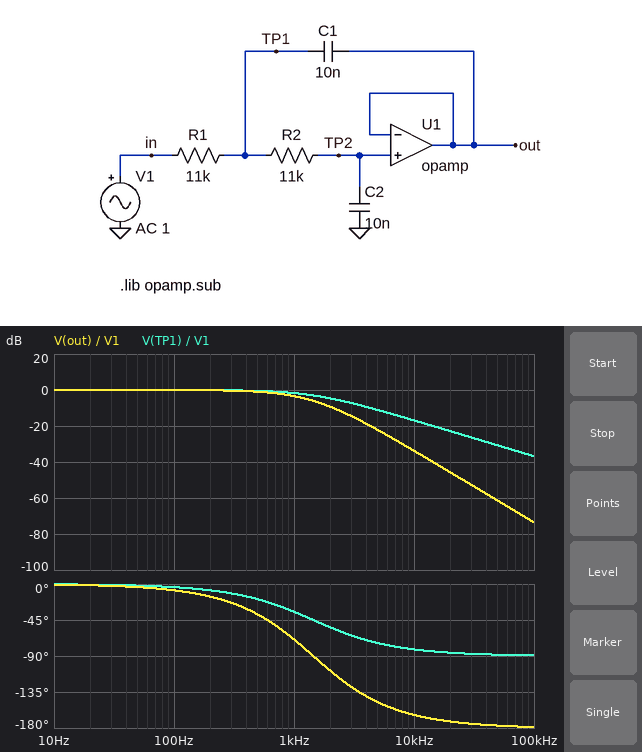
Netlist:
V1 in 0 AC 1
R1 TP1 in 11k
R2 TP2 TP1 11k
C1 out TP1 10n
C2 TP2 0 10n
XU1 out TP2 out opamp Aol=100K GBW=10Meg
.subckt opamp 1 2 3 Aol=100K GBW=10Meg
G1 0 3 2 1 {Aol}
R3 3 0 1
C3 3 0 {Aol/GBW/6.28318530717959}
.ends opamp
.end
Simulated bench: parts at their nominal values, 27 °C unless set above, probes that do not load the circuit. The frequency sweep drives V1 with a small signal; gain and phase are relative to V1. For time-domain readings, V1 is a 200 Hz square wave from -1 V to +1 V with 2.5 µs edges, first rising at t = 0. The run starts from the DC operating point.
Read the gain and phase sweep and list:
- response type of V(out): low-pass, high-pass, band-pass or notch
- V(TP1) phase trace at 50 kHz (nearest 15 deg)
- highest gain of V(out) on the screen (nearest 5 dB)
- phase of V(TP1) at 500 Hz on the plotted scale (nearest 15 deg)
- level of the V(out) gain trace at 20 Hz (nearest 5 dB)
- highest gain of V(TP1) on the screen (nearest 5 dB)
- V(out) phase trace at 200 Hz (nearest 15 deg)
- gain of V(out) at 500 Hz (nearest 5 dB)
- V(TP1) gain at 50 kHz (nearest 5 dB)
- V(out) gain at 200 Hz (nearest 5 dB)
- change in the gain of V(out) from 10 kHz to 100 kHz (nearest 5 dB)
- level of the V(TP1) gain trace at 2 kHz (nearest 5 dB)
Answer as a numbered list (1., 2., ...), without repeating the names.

1. low-pass
2. -90 deg
3. 0 dB
4. -15 deg
5. 0 dB
6. 0 dB
7. -15 deg
8. 0 dB
9. -30 dB
10. 0 dB
11. -40 dB
12. -5 dB
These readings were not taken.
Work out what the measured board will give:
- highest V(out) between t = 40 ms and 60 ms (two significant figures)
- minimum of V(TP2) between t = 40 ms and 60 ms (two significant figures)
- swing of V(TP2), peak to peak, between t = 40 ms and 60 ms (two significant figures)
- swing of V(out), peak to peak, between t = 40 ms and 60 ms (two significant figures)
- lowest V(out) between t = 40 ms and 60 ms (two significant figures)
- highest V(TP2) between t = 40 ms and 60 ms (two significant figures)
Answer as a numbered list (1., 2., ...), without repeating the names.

1. 1.0 V
2. -1.0 V
3. 2.0 V
4. 2.0 V
5. -1.0 V
6. 1.0 V
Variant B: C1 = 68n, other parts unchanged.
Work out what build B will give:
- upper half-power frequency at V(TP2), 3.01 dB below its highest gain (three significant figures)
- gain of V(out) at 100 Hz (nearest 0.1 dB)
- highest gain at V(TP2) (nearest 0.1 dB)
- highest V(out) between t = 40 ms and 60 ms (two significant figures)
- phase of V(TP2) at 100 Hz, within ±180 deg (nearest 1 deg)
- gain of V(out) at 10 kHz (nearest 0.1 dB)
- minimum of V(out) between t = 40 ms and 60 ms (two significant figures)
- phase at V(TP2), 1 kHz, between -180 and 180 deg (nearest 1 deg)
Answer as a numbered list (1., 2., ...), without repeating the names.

1. 660 Hz
2. 0.2 dB
3. 3.0 dB
4. 1.5 V
5. -8 deg
6. -50.2 dB
7. -1.5 V
8. -148 deg
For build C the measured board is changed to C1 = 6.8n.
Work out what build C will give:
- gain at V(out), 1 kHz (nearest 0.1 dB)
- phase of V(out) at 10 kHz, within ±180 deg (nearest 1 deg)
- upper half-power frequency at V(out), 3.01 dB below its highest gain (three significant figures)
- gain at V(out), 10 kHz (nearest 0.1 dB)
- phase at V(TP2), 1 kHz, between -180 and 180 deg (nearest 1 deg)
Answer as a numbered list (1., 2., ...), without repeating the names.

1. -3.7 dB
2. -156 deg
3. 864 Hz
4. -30.7 dB
5. -64 deg
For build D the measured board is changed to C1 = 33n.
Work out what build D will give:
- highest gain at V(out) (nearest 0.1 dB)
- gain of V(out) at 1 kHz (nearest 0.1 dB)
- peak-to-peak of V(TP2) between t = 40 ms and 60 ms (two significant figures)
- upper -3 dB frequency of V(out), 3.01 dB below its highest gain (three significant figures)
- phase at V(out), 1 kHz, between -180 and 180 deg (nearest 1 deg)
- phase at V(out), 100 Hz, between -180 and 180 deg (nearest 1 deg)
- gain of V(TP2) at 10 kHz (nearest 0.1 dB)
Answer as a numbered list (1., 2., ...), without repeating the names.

1. 0.7 dB
2. -3.5 dB
3. 2.5 V
4. 913 Hz
5. -113 deg
6. -8 deg
7. -43.9 dB
